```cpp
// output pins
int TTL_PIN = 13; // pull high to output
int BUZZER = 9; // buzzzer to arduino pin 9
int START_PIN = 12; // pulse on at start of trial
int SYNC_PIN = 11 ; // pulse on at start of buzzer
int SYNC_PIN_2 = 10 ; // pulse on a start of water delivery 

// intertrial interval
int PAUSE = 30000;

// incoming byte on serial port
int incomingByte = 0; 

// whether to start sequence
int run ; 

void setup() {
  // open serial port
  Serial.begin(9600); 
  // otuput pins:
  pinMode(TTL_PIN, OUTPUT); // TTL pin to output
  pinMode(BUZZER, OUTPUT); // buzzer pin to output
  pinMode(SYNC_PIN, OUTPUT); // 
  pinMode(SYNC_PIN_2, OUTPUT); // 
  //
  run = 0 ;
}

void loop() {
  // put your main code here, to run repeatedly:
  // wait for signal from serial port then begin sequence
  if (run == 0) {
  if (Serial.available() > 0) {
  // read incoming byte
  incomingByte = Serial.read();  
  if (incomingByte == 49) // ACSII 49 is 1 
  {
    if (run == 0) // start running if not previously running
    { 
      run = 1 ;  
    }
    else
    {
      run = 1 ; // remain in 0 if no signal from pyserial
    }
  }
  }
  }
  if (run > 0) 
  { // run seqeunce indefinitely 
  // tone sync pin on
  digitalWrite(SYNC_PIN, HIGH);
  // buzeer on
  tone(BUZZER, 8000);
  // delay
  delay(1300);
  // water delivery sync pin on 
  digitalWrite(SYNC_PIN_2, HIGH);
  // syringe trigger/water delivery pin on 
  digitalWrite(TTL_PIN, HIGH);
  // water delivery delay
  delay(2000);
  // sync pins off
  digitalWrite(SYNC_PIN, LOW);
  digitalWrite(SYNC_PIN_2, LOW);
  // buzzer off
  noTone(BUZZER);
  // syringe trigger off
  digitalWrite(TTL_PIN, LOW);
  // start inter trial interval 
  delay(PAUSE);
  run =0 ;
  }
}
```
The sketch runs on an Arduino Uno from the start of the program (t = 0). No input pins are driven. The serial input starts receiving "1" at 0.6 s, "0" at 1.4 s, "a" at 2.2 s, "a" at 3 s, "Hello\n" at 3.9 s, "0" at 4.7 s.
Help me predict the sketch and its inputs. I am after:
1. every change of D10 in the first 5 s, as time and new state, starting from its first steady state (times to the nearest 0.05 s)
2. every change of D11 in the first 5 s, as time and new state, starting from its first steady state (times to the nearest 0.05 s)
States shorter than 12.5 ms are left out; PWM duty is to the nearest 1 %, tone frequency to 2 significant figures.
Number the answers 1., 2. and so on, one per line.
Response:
1. 0 s low; 1.9 s high; 3.9 s low
2. 0 s low; 0.6 s high; 3.9 s low
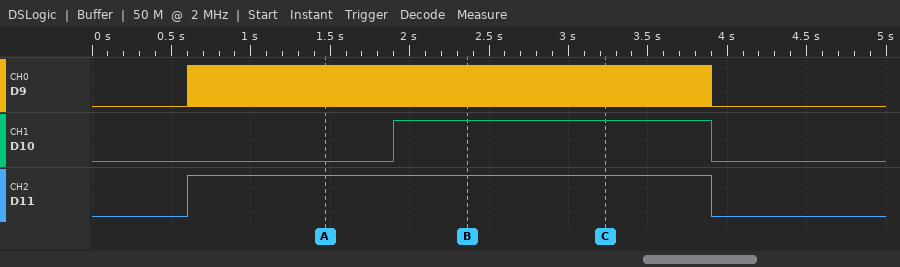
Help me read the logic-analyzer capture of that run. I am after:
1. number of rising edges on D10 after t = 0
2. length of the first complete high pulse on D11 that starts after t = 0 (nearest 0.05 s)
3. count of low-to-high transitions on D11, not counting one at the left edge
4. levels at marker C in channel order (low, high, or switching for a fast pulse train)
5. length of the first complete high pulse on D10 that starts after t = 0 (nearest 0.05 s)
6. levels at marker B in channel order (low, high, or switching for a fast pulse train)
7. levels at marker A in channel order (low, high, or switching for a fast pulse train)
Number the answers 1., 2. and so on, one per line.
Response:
1. 1
2. 3.30 s
3. 1
4. D9 switching, D10 high, D11 high
5. 2.00 s
6. D9 switching, D10 high, D11 high
7. D9 switching, D10 low, D11 high
